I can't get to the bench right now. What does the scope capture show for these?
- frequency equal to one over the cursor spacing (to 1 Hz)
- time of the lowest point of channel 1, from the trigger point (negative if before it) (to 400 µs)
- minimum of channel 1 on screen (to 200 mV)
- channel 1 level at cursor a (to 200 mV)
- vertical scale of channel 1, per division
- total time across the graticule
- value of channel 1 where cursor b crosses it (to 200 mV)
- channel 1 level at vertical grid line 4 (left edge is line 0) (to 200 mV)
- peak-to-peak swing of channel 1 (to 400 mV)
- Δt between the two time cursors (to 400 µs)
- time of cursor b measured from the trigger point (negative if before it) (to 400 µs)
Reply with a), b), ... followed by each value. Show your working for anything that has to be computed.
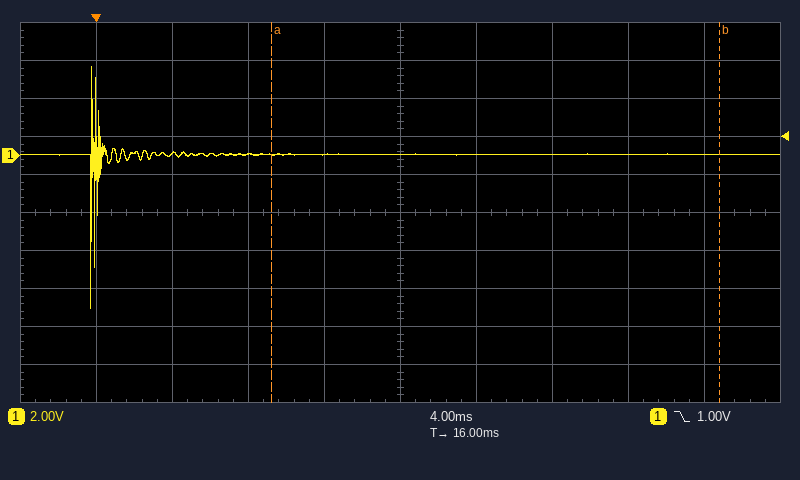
a) 1 / 23.6 ms ≈ 42 Hz
b) -400 µs
c) -8.0 V
d) 0.0 V
e) 2 V
f) 40 ms
g) 0.0 V
h) 0.0 V
i) 12.8 V
j) 23.6 ms
k) +32.8 ms
